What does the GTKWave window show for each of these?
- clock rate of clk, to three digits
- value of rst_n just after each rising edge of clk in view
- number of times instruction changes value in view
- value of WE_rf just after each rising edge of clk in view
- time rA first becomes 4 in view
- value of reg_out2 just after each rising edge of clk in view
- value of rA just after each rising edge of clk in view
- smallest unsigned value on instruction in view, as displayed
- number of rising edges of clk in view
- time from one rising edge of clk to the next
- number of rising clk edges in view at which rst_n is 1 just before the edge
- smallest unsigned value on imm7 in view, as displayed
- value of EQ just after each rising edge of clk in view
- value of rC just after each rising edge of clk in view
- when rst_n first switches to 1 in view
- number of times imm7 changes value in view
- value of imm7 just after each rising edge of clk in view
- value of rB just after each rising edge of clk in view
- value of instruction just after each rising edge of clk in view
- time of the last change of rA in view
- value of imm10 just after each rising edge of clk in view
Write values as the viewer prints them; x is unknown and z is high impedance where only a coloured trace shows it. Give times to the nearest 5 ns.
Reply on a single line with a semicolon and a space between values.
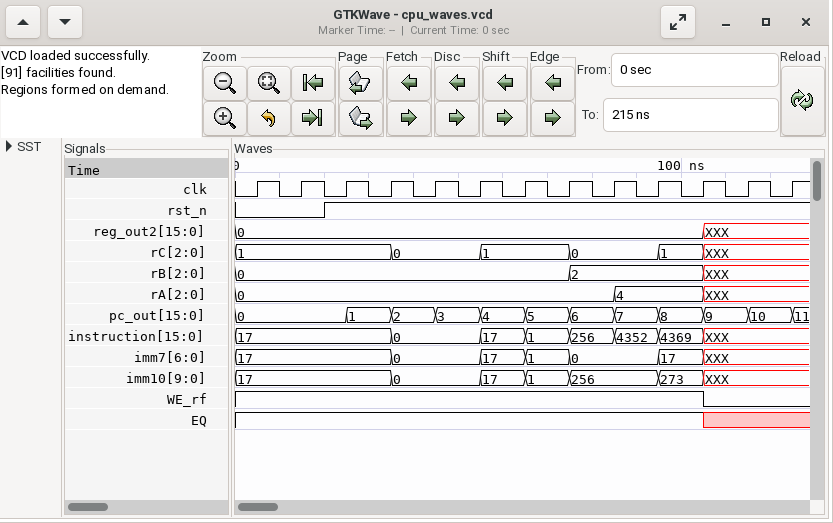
100 MHz; 0 0 1 1 1 1 1 1 1 1 1 1 1; 7; 1 1 1 1 1 1 1 1 1 1 0 0 0; 85 ns; 0, 0, 0, 0, 0, 0, 0, 0, 0, 0, XXX, XXX, XXX; 0, 0, 0, 0, 0, 0, 0, 0, 4, 4, XXX, XXX, XXX; 0; 13; 10 ns; 11; 0; 1 1 1 1 1 1 1 1 1 1 x x x; 1, 1, 1, 0, 0, 1, 1, 0, 0, 1, XXX, XXX, XXX; 20 ns; 6; 17, 17, 17, 0, 0, 17, 1, 0, 0, 17, XXX, XXX, XXX; 0, 0, 0, 0, 0, 0, 0, 2, 2, 2, XXX, XXX, XXX; 17, 17, 17, 0, 0, 17, 1, 256, 4352, 4369, XXX, XXX, XXX; 105 ns; 17, 17, 17, 0, 0, 17, 1, 256, 256, 273, XXX, XXX, XXX
